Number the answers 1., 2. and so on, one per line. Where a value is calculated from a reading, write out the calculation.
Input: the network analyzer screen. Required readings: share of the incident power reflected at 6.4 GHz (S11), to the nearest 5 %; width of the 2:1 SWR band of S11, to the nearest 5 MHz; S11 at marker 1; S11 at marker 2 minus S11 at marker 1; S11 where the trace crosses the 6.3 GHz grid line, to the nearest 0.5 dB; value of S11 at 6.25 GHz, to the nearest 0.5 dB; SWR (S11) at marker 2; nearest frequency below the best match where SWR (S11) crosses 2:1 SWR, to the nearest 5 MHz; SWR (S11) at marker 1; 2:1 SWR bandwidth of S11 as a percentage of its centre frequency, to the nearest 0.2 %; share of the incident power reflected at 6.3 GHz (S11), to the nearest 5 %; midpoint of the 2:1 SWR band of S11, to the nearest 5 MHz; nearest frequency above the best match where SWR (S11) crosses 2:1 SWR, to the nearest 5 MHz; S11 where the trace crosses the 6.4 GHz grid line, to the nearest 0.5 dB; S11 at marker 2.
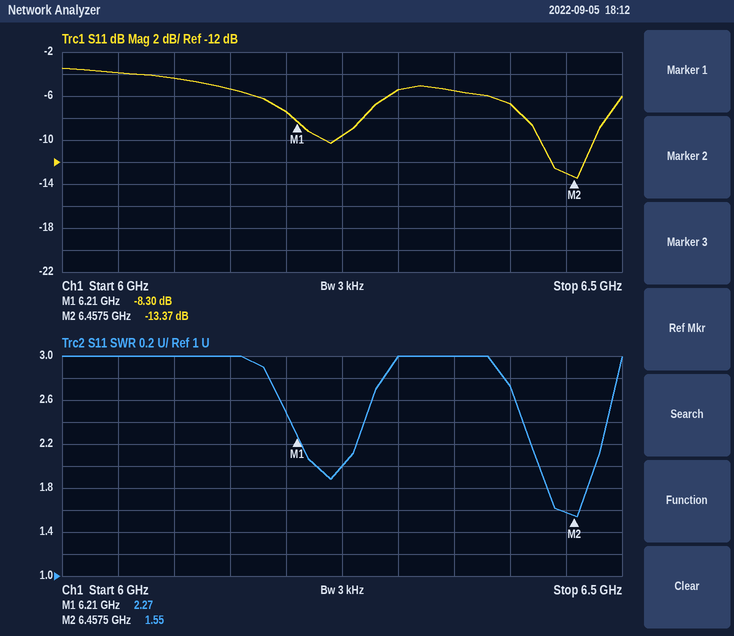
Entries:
1. 10^(-6.5/10) ≈ 22.4 %, so 20 % to the nearest 5 %
2. 6.475 GHz − 6.425 GHz = 50 MHz
3. -8.30 dB
4. -13.37 − (-8.3) = -5.07 dB
5. -5.5 dB
6. -9.5 dB
7. 1.55
8. 6.425 GHz
9. 2.27
10. 50 MHz / 6.45 GHz ≈ 0.8 %
11. 10^(-5.5/10) ≈ 28.2 %, so 30 % to the nearest 5 %
12. 6.450 GHz
13. 6.475 GHz
14. -6.5 dB
15. -13.37 dB
